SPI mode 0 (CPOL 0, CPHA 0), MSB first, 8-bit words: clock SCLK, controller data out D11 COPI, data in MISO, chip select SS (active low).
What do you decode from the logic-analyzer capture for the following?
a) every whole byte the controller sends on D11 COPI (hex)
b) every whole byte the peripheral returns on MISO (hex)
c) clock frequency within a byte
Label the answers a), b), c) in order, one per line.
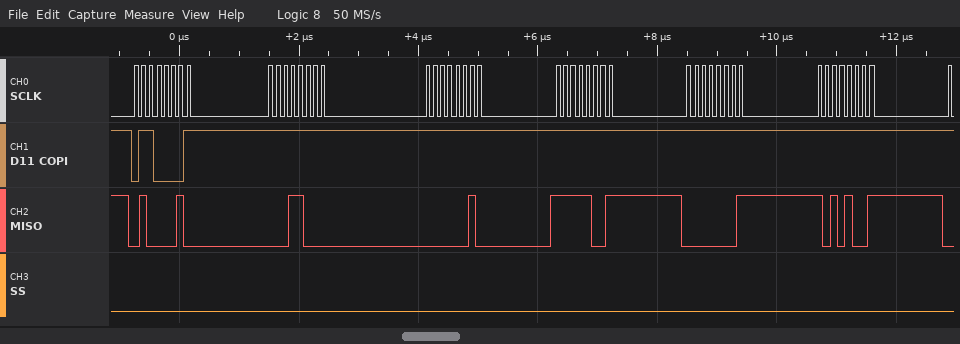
a) 61 FF FF FF FF FF
b) 42 18 02 F9 01 A9
c) 8 MHz
